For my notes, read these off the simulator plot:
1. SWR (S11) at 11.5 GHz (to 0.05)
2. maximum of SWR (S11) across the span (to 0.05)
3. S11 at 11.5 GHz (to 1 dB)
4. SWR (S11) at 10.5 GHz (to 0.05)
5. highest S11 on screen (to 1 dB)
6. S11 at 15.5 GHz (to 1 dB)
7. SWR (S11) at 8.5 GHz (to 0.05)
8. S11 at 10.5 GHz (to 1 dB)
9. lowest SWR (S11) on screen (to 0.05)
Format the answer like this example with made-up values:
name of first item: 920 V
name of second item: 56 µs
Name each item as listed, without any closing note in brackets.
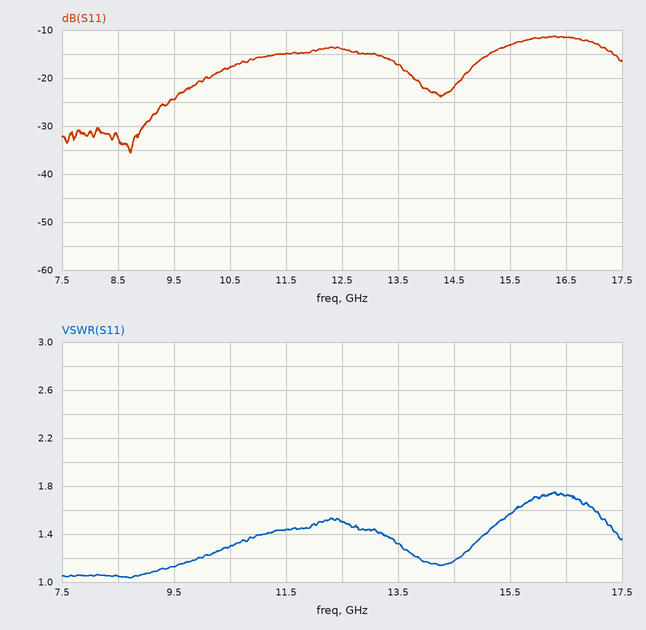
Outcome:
SWR (S11) at 11.5 GHz: 1.45
maximum of SWR (S11) across the span: 1.75
S11 at 11.5 GHz: -15 dB
SWR (S11) at 10.5 GHz: 1.30
highest S11 on screen: -11 dB
S11 at 15.5 GHz: -13 dB
SWR (S11) at 8.5 GHz: 1.05
S11 at 10.5 GHz: -18 dB
lowest SWR (S11) on screen: 1.05
